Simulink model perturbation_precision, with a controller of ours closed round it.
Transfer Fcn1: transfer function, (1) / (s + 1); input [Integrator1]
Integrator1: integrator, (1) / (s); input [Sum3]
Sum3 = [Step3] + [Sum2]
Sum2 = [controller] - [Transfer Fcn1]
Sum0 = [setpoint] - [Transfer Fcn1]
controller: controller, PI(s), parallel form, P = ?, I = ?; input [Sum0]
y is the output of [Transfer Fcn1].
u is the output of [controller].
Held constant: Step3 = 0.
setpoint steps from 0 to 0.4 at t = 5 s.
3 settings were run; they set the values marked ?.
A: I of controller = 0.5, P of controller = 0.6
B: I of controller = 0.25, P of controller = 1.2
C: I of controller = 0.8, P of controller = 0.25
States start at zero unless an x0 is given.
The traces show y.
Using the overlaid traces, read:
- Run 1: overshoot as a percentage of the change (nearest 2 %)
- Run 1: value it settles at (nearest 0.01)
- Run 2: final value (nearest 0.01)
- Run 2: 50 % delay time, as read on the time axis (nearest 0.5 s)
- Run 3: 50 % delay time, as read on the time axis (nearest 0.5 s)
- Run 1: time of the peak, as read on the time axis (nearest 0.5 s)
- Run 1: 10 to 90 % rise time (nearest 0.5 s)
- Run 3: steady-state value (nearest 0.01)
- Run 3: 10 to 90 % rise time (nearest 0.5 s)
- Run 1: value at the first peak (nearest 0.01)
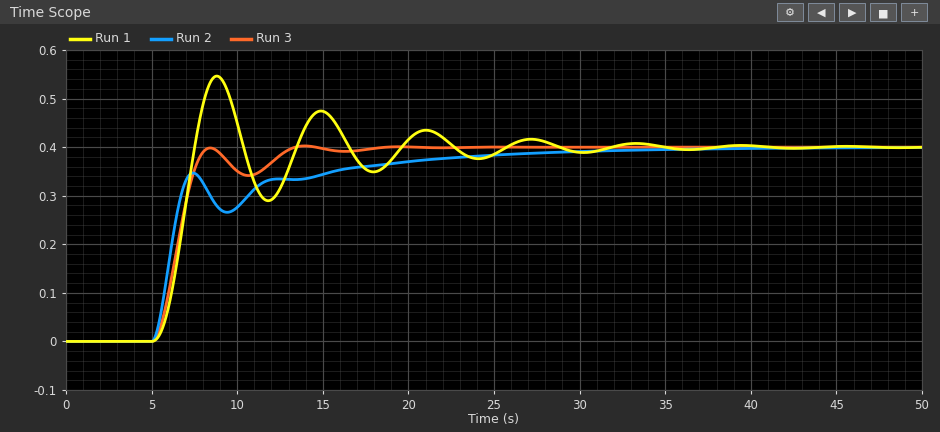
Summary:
36 %
0.40
0.40
6.0 s
6.5 s
9.0 s
1.5 s
0.40
2.0 s
0.55
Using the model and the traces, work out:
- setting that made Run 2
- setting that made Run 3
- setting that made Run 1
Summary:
B
A
C
